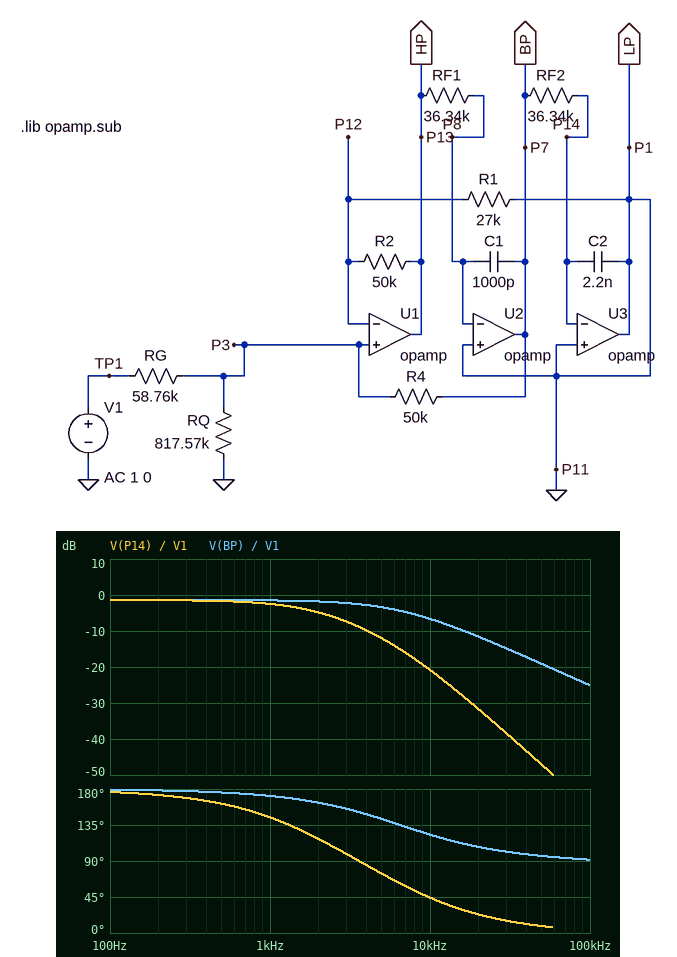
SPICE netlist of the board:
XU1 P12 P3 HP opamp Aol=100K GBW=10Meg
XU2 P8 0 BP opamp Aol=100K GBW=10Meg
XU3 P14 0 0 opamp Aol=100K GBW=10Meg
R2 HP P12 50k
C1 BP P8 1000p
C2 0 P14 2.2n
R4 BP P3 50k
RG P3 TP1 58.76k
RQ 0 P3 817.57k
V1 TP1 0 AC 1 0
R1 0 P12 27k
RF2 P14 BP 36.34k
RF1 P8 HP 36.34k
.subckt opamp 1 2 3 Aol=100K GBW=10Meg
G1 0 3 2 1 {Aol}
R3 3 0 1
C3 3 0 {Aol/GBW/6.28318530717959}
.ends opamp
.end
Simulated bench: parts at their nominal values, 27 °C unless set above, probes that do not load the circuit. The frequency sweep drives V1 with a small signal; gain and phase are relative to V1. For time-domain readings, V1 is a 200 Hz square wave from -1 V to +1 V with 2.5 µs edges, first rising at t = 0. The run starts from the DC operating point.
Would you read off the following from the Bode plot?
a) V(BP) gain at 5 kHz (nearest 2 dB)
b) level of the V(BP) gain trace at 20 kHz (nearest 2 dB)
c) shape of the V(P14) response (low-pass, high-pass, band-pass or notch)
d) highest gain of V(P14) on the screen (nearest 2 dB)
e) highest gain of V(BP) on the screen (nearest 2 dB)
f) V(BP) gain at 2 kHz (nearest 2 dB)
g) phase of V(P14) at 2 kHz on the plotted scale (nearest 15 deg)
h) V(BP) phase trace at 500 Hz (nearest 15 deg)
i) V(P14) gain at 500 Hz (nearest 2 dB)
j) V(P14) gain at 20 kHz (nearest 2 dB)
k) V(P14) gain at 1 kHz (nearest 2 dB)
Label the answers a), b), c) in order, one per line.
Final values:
a) -4 dB
b) -12 dB
c) low-pass
d) -2 dB
e) -2 dB
f) -2 dB
g) 120 deg
h) 180 deg
i) -2 dB
j) -32 dB
k) -2 dB
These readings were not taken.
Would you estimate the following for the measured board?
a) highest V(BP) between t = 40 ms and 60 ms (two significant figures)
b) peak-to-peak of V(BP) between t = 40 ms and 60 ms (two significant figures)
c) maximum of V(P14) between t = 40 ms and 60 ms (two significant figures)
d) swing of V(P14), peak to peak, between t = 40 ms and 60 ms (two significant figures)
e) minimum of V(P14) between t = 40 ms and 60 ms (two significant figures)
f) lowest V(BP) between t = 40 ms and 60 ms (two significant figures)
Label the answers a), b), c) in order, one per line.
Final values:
a) 850 mV
b) 1.7 V
c) 850 mV
d) 1.7 V
e) -850 mV
f) -850 mV
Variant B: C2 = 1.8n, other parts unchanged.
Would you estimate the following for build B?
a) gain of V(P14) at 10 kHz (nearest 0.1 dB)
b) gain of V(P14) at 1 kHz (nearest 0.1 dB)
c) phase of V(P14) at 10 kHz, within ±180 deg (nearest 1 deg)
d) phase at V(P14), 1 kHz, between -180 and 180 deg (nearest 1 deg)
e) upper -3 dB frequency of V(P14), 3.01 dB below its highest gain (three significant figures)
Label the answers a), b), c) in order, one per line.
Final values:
a) -19.2 dB
b) -2.2 dB
c) 47 deg
d) 149 deg
e) 2.18 kHz
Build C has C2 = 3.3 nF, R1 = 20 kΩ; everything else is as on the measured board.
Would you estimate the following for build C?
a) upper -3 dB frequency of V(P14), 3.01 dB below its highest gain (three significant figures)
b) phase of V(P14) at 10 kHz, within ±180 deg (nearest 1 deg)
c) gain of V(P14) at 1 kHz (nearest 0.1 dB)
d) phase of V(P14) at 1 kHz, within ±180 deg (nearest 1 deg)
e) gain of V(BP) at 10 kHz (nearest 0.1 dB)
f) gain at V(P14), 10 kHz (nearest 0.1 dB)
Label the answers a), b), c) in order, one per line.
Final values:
a) 1.29 kHz
b) 46 deg
c) -3.4 dB
d) 136 deg
e) -5.5 dB
f) -23.1 dB
